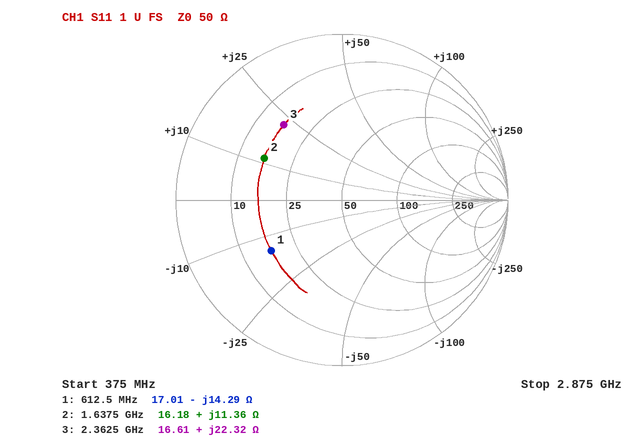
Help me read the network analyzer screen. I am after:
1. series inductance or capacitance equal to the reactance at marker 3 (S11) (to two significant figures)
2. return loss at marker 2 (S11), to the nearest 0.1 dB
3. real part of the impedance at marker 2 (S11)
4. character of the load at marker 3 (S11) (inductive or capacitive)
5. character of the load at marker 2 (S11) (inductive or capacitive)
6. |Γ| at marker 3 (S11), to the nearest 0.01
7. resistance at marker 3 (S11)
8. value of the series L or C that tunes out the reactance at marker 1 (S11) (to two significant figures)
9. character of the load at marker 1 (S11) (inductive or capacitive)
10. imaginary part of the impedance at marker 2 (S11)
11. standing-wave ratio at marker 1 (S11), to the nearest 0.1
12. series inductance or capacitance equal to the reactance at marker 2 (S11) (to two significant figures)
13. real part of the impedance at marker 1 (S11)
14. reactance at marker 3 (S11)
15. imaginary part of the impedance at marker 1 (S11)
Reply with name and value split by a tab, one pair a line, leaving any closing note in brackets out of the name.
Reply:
series inductance or capacitance equal to the reactance at marker 3 (S11)	1.5 nH
return loss at marker 2 (S11), to the nearest 0.1 dB	5.5 dB
real part of the impedance at marker 2	16.18 Ω
character of the load at marker 3 (S11)	inductive
character of the load at marker 2 (S11)	inductive
|Γ| at marker 3 (S11), to the nearest 0.01	0.57
resistance at marker 3	16.61 Ω
value of the series L or C that tunes out the reactance at marker 1 (S11)	3.7 nH
character of the load at marker 1 (S11)	capacitive
imaginary part of the impedance at marker 2	+11.36 Ω
standing-wave ratio at marker 1 (S11), to the nearest 0.1	3.2
series inductance or capacitance equal to the reactance at marker 2 (S11)	1.1 nH
real part of the impedance at marker 1	17.01 Ω
reactance at marker 3	+22.32 Ω
imaginary part of the impedance at marker 1	-14.29 Ω
